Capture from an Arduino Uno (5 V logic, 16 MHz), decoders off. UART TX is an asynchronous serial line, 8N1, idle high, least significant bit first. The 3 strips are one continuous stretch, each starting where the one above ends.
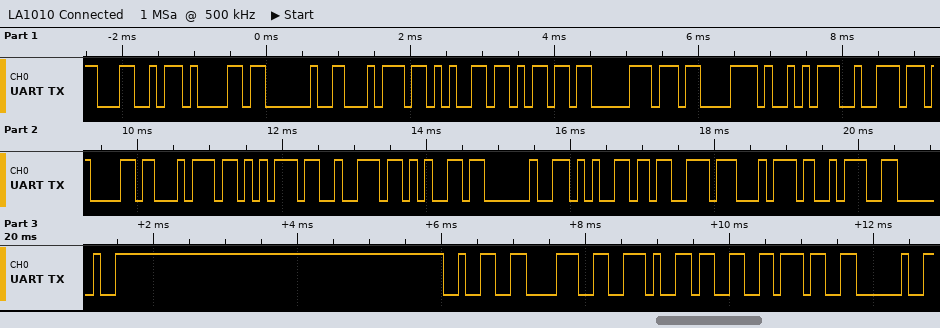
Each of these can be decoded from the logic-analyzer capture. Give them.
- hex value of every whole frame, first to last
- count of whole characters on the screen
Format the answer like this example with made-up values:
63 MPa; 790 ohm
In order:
4C 61 20 74 65 6D 70 C3 A9 72 61 74 75 72 65 20 65 73 74 3A 20 32 38 2E 33 37 20; 27
